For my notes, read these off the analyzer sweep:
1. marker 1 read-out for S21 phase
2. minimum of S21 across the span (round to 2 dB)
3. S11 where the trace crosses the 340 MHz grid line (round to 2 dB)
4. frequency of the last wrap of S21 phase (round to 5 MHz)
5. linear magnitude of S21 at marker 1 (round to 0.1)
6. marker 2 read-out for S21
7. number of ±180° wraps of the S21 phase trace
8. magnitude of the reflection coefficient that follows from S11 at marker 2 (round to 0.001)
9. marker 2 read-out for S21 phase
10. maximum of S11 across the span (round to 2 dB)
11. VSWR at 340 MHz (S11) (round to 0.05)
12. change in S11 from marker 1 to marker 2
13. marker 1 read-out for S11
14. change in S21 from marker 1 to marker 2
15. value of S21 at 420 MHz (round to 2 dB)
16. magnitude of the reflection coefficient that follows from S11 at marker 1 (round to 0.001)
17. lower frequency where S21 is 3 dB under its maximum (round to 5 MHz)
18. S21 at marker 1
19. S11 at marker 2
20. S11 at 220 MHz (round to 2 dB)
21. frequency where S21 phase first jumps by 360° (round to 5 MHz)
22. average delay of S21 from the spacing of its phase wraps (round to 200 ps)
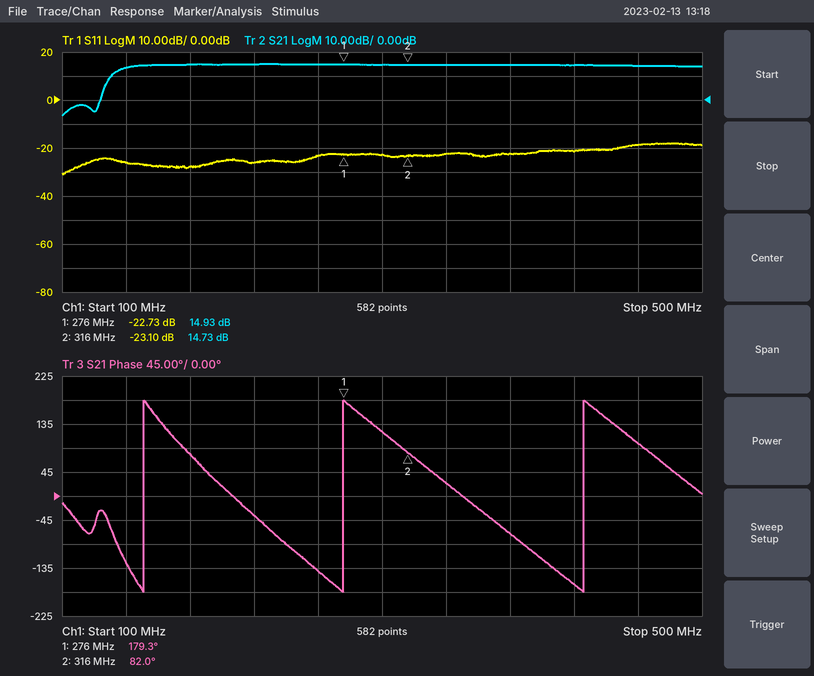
179.3°
-6 dB
-22 dB
425 MHz
5.6
14.73 dB
3
0.070
82.0°
-18 dB
1.15
-0.37 dB
-22.73 dB
-0.20 dB
14 dB
0.073
135 MHz
14.93 dB
-23.10 dB
-26 dB
150 MHz
7.2 ns
